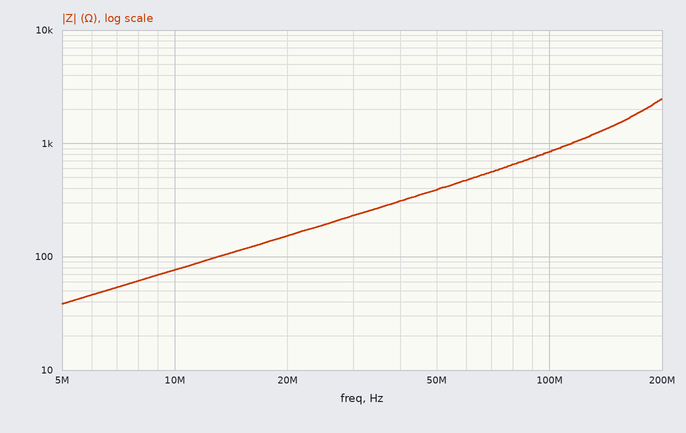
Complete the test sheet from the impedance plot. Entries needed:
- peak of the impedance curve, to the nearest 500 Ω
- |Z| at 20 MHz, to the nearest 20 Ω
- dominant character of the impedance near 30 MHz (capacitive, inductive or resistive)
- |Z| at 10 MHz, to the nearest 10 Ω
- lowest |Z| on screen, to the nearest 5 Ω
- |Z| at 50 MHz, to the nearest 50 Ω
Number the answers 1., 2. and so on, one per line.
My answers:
1. 2.5 kΩ
2. 160 Ω
3. inductive
4. 80 Ω
5. 40 Ω
6. 400 Ω
